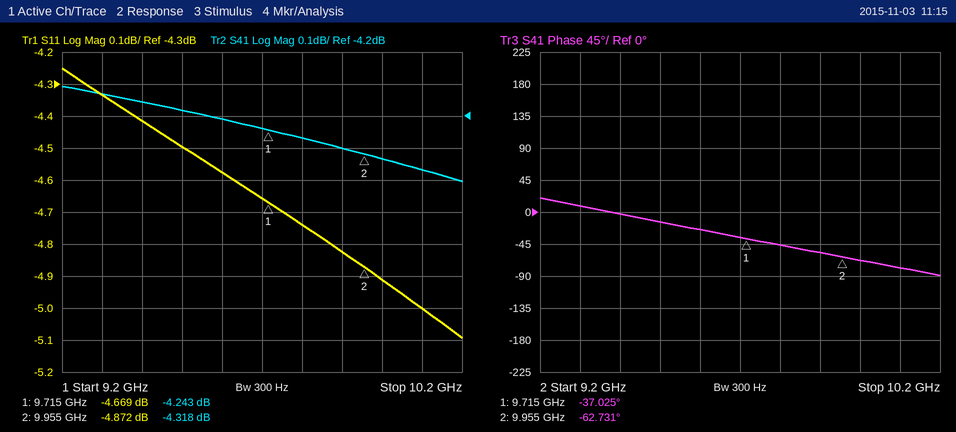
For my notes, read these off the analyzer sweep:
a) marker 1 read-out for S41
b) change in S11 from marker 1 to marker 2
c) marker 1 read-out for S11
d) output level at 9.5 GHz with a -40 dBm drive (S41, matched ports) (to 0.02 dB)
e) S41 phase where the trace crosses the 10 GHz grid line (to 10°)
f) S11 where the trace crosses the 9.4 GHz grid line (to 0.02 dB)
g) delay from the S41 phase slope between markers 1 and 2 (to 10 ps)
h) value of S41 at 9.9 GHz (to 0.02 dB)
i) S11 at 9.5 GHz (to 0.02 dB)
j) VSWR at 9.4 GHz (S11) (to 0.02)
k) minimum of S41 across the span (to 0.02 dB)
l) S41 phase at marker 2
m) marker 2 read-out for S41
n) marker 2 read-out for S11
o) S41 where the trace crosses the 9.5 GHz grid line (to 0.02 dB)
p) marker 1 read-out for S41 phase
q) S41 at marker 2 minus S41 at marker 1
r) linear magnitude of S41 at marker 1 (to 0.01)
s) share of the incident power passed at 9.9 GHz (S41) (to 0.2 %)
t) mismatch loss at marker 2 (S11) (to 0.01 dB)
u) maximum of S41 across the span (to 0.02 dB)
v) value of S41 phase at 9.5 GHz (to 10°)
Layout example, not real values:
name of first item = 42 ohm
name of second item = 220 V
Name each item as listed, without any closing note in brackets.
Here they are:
marker 1 read-out for S41 = -4.243 dB
change in S11 from marker 1 to marker 2 = -0.203 dB
marker 1 read-out for S11 = -4.669 dB
output level at 9.5 GHz with a -40 dBm drive (S41, matched ports) = -44.18 dBm
S41 phase where the trace crosses the 10 GHz grid line = -70°
S11 where the trace crosses the 9.4 GHz grid line = -4.42 dB
delay from the S41 phase slope between markers 1 and 2 = 300 ps
value of S41 at 9.9 GHz = -4.30 dB
S11 at 9.5 GHz = -4.50 dB
VSWR at 9.4 GHz (S11) = 4.02
minimum of S41 across the span = -4.40 dB
S41 phase at marker 2 = -62.731°
marker 2 read-out for S41 = -4.318 dB
marker 2 read-out for S11 = -4.872 dB
S41 where the trace crosses the 9.5 GHz grid line = -4.18 dB
marker 1 read-out for S41 phase = -37.025°
S41 at marker 2 minus S41 at marker 1 = -0.075 dB
linear magnitude of S41 at marker 1 = 0.61
share of the incident power passed at 9.9 GHz (S41) = 37.2 %
mismatch loss at marker 2 (S11) = 1.71 dB
maximum of S41 across the span = -4.10 dB
value of S41 phase at 9.5 GHz = -10°
